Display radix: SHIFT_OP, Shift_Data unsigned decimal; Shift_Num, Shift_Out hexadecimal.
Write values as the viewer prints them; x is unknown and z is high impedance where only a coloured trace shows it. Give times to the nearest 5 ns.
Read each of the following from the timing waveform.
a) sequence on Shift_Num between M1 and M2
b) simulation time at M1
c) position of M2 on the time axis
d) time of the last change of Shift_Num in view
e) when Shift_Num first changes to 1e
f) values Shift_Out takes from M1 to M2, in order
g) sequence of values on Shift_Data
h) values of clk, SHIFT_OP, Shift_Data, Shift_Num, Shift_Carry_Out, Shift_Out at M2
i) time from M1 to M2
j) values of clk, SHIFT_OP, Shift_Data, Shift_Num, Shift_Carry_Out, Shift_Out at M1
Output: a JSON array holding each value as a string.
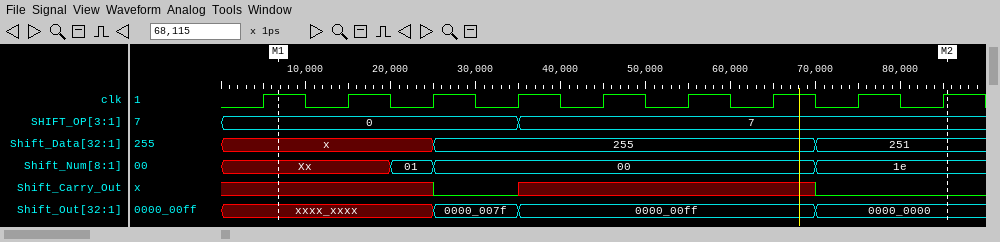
["Xx, 01, 00, 1e", "5 ns", "85 ns", "70 ns", "70 ns", "xxxx_xxxx, 0000_007f, 0000_00ff, 0000_0000", "x, 255, 251", "clk=1, SHIFT_OP=7, Shift_Data=251, Shift_Num=1e, Shift_Carry_Out=0, Shift_Out=0000_0000", "80 ns", "clk=1, SHIFT_OP=0, Shift_Data=x, Shift_Num=Xx, Shift_Carry_Out=x, Shift_Out=xxxx_xxxx"]
